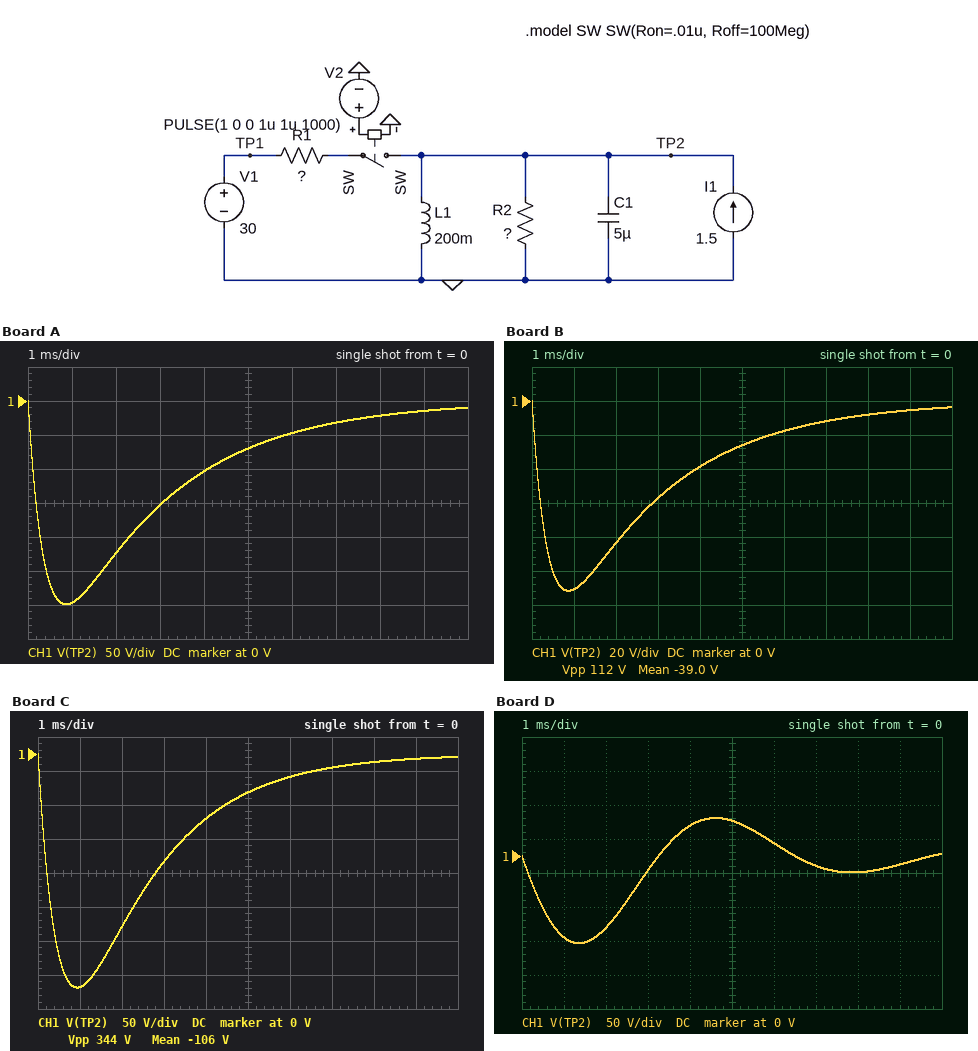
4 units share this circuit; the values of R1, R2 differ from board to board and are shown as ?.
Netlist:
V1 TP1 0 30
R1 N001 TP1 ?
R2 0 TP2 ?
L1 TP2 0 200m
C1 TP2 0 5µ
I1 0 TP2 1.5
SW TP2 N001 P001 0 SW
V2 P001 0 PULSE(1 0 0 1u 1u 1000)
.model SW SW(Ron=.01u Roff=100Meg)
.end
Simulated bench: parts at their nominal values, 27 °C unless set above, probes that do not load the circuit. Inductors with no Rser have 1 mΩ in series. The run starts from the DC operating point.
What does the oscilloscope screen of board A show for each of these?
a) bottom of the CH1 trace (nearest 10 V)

-300 V
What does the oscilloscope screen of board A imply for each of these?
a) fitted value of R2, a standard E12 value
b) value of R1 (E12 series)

68 Ω
5.6 Ω
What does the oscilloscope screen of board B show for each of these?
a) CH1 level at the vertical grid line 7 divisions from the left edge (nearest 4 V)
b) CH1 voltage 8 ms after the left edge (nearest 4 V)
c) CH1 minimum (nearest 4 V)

-12 V
-8 V
-112 V
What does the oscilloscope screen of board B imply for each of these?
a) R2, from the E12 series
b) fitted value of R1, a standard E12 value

68 Ω
15 Ω
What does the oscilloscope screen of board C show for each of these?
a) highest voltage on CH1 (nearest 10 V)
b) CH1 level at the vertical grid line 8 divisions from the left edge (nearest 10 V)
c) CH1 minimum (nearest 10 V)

0 V
-10 V
-340 V
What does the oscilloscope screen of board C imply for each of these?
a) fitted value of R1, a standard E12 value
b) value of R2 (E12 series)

5.6 Ω
82 Ω
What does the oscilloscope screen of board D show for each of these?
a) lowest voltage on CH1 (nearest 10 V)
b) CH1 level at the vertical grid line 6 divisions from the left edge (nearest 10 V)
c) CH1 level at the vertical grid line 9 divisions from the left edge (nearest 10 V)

-130 V
20 V
-10 V
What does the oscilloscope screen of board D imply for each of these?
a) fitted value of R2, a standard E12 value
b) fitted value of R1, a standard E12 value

390 Ω
33 Ω
